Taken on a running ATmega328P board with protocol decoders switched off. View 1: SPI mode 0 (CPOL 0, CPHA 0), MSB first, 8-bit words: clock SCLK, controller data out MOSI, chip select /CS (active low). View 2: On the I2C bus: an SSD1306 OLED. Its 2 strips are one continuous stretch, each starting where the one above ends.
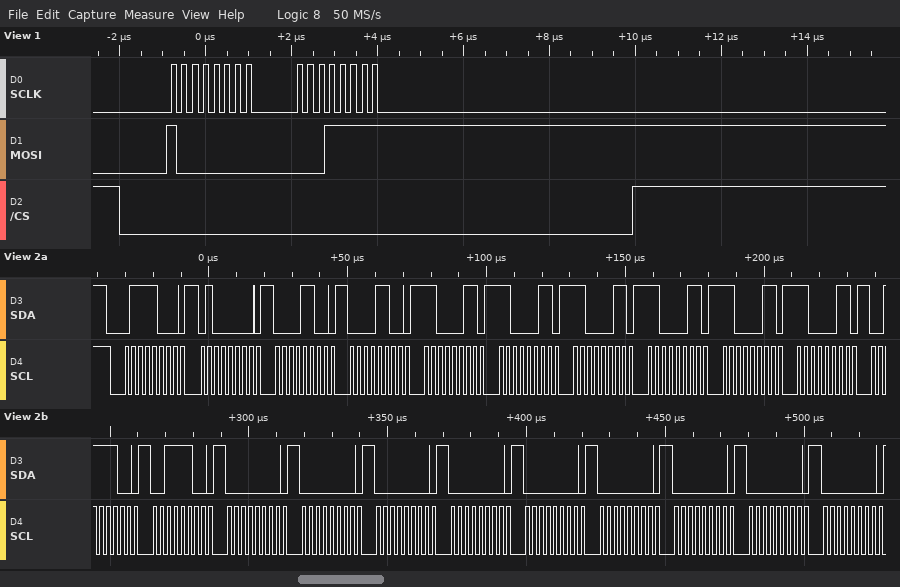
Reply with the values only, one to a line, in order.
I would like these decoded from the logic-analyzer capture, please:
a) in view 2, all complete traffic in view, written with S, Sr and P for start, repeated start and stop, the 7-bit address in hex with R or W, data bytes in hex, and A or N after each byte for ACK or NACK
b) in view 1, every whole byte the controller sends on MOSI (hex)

S 3CW A 40 A 0C A 0C A C3 A C3 A C3 A C3 A C3 A C3 A 3C A 3C A 00 A 00 A 00 A 00 A 00 A 00 A 00 A 00 A 00 A
80 1F
